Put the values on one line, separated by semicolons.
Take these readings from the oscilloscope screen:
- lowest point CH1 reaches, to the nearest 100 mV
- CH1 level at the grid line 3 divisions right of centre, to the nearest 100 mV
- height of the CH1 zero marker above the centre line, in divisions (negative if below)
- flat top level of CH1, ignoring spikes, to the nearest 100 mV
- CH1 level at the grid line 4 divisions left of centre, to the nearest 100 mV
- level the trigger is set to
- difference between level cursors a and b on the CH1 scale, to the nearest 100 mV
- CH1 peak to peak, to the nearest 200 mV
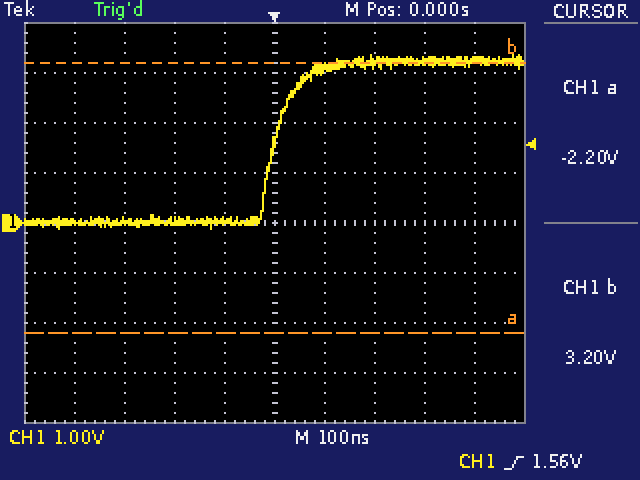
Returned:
-100 mV; 3.2 V; 0.0 div; 3.2 V; 0.0 V; 1.56 V; 5.4 V; 3.4 V
